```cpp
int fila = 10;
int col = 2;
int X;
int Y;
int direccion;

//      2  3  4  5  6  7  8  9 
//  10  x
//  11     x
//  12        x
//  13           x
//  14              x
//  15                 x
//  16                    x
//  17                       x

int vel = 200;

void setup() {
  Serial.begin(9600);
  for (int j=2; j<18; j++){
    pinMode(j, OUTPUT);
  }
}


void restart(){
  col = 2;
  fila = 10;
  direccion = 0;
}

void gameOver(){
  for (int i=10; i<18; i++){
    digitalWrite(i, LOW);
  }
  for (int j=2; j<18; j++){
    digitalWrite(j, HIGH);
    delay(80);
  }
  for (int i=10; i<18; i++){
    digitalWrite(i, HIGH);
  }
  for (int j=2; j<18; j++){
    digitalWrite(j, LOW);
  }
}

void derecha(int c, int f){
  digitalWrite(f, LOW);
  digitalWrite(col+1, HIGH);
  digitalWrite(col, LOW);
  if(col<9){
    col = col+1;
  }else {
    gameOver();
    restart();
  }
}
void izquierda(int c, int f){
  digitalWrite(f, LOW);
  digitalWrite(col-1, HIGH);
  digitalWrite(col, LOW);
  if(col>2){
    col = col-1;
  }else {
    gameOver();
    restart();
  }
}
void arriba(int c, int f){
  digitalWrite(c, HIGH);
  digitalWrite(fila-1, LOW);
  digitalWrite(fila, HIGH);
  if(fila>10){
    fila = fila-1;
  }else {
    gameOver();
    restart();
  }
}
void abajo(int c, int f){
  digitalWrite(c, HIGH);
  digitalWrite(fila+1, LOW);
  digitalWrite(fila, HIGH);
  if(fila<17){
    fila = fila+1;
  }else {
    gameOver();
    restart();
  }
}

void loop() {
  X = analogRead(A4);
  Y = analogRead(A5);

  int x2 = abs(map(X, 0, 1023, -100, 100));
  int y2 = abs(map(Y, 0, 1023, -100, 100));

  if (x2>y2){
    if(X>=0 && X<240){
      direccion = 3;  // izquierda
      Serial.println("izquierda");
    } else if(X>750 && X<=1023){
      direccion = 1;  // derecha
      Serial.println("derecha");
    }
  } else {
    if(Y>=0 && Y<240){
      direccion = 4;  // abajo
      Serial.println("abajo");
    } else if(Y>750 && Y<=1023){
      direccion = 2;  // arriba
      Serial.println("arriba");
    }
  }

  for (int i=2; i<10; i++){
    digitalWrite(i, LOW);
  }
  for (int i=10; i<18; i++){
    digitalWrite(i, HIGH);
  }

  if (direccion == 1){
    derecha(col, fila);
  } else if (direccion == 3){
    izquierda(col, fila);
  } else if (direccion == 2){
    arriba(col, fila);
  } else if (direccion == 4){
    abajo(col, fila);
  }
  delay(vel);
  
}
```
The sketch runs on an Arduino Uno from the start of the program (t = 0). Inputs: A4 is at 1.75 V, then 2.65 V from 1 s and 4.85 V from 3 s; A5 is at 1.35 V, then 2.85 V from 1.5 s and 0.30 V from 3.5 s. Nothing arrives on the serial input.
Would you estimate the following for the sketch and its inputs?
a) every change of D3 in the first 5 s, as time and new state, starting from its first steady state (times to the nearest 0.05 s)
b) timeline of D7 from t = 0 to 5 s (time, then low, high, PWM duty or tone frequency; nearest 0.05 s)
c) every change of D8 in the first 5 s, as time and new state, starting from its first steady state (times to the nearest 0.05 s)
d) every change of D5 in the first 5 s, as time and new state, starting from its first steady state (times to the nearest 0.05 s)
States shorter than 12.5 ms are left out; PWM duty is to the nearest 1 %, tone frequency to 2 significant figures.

0 s low; 3 s high; 3.2 s low; 4.5 s high
0 s low; 3.8 s high; 4 s low; 4.8 s high
0 s low; 4 s high; 4.2 s low; 4.9 s high
0 s low; 3.4 s high; 3.6 s low; 4.65 s high
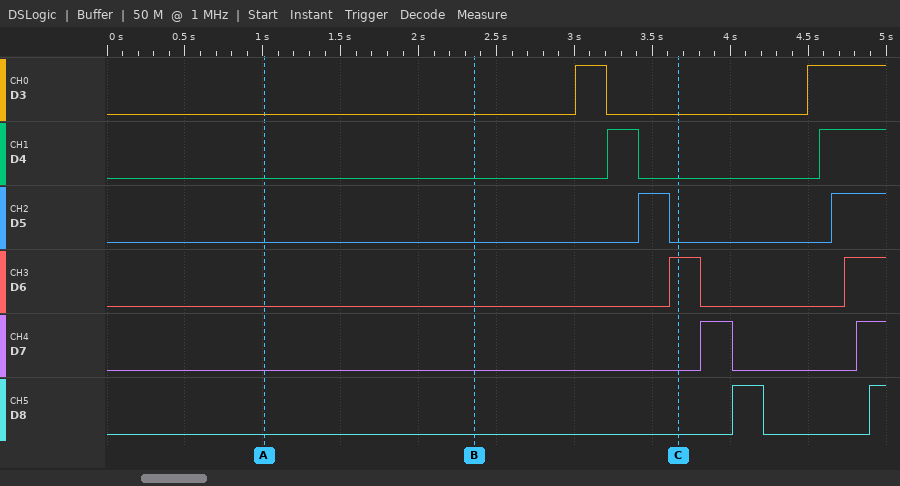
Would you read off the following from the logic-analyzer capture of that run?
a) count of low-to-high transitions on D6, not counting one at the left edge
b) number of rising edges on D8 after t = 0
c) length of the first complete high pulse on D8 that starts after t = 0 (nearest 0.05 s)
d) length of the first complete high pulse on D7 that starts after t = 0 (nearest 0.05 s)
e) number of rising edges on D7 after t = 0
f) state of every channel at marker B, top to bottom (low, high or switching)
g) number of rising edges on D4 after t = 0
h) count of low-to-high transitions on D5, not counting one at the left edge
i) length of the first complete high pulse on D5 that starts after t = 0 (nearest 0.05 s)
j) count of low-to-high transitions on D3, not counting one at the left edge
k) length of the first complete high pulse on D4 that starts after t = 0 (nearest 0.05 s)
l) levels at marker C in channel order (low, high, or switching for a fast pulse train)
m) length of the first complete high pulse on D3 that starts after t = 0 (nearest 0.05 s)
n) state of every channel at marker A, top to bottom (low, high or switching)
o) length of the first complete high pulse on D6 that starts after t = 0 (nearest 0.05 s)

2
2
0.20 s
0.20 s
2
D3 low, D4 low, D5 low, D6 low, D7 low, D8 low
2
2
0.20 s
2
0.20 s
D3 low, D4 low, D5 low, D6 high, D7 low, D8 low
0.20 s
D3 low, D4 low, D5 low, D6 low, D7 low, D8 low
0.20 s
